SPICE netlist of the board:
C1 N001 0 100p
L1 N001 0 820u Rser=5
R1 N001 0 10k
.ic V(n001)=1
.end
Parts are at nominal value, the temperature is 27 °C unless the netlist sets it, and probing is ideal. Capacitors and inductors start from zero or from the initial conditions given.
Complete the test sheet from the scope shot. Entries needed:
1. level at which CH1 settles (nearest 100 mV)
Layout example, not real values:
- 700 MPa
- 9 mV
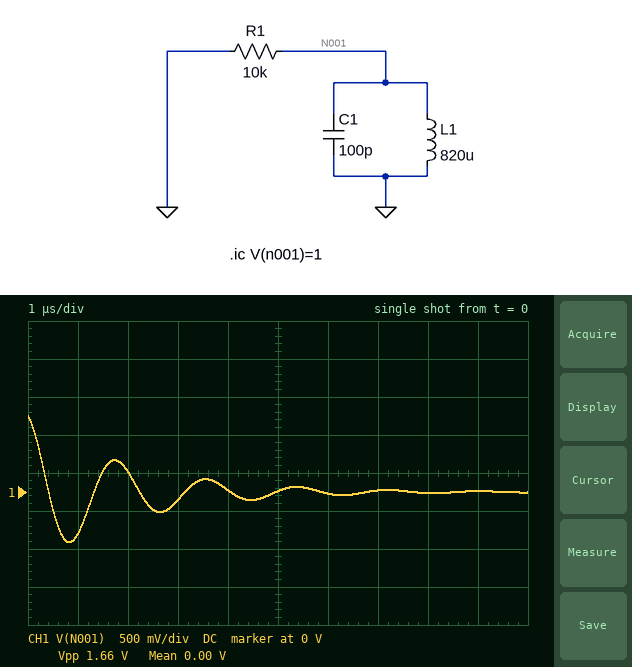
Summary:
- 0 V
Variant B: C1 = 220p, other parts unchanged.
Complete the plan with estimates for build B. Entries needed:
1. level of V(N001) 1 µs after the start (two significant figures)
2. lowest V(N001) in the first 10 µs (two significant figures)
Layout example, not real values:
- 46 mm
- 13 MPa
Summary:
- -610 mV
- -750 mV
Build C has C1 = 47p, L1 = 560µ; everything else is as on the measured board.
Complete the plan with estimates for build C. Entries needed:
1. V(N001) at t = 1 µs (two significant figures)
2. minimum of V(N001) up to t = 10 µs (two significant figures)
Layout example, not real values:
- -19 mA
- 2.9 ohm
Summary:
- 350 mV
- -610 mV
